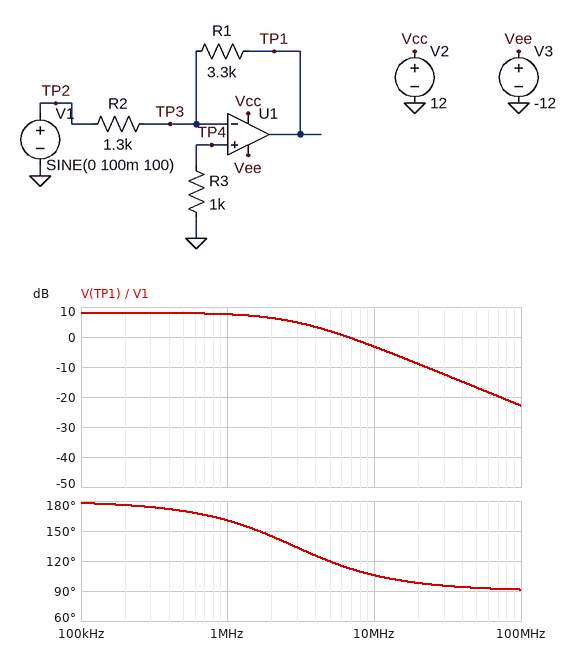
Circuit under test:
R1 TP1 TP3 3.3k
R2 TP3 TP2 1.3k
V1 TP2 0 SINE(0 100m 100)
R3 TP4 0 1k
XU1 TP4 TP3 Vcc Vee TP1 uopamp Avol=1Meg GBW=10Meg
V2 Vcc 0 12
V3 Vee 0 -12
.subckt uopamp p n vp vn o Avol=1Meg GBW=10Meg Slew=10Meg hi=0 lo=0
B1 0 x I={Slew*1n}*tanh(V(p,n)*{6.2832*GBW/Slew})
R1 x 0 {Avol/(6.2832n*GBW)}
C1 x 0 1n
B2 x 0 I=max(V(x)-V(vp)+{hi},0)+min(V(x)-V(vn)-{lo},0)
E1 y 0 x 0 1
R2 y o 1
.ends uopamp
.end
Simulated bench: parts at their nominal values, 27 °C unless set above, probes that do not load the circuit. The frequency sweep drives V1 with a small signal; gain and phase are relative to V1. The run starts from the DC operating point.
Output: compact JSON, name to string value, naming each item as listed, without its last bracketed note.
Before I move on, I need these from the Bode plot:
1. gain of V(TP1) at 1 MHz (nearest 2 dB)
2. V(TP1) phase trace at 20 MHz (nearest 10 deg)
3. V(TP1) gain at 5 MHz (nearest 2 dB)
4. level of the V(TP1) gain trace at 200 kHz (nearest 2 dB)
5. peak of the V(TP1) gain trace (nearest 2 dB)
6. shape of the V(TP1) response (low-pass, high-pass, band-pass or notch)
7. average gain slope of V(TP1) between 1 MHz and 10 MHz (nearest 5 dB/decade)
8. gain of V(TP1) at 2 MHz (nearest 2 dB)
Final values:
{"gain of V(TP1) at 1 MHz": "8 dB", "V(TP1) phase trace at 20 MHz": "100 deg", "V(TP1) gain at 5 MHz": "2 dB", "level of the V(TP1) gain trace at 200 kHz": "8 dB", "peak of the V(TP1) gain trace": "8 dB", "shape of the V(TP1) response": "low-pass", "average gain slope of V(TP1) between 1 MHz and 10 MHz": "-10 dB/decade", "gain of V(TP1) at 2 MHz": "6 dB"}
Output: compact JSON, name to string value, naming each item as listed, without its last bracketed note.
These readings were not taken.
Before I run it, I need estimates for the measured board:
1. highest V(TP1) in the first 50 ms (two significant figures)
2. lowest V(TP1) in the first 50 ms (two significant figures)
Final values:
{"highest V(TP1) in the first 50 ms": "250 mV", "lowest V(TP1) in the first 50 ms": "-250 mV"}
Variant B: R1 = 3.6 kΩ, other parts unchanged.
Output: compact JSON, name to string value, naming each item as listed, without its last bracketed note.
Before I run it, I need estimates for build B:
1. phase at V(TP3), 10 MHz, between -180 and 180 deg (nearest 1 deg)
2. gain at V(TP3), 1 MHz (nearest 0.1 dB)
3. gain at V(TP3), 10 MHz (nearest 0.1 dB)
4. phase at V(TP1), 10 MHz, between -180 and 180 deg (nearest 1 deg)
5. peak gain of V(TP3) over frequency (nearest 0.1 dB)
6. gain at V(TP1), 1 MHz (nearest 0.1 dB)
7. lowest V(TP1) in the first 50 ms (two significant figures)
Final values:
{"phase at V(TP3), 10 MHz, between -180 and 180 deg": "15 deg", "gain at V(TP3), 1 MHz": "-11.7 dB", "gain at V(TP3), 10 MHz": "-3.0 dB", "phase at V(TP1), 10 MHz, between -180 and 180 deg": "105 deg", "peak gain of V(TP3) over frequency": "-2.7 dB", "gain at V(TP1), 1 MHz": "8.3 dB", "lowest V(TP1) in the first 50 ms": "-280 mV"}
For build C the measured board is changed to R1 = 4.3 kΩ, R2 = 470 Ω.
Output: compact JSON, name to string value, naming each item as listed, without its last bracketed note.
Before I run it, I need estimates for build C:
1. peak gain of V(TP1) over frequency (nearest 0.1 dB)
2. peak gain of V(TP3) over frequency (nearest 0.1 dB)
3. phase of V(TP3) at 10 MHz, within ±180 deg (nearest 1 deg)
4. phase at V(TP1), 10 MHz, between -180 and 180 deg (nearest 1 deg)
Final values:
{"peak gain of V(TP1) over frequency": "19.2 dB", "peak gain of V(TP3) over frequency": "-0.9 dB", "phase of V(TP3) at 10 MHz, within ±180 deg": "6 deg", "phase at V(TP1), 10 MHz, between -180 and 180 deg": "96 deg"}
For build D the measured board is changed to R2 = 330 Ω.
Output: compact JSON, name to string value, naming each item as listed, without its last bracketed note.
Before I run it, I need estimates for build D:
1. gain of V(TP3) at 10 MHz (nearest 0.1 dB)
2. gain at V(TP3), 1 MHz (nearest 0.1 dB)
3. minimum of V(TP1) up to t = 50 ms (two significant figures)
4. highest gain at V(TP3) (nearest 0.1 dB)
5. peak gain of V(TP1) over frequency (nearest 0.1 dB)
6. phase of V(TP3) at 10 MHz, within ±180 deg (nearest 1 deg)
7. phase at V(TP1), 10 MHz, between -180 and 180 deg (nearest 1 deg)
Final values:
{"gain of V(TP3) at 10 MHz": "-0.9 dB", "gain at V(TP3), 1 MHz": "-3.4 dB", "minimum of V(TP1) up to t = 50 ms": "-1.0 V", "highest gain at V(TP3)": "-0.8 dB", "peak gain of V(TP1) over frequency": "20.0 dB", "phase of V(TP3) at 10 MHz, within ±180 deg": "5 deg", "phase at V(TP1), 10 MHz, between -180 and 180 deg": "95 deg"}
